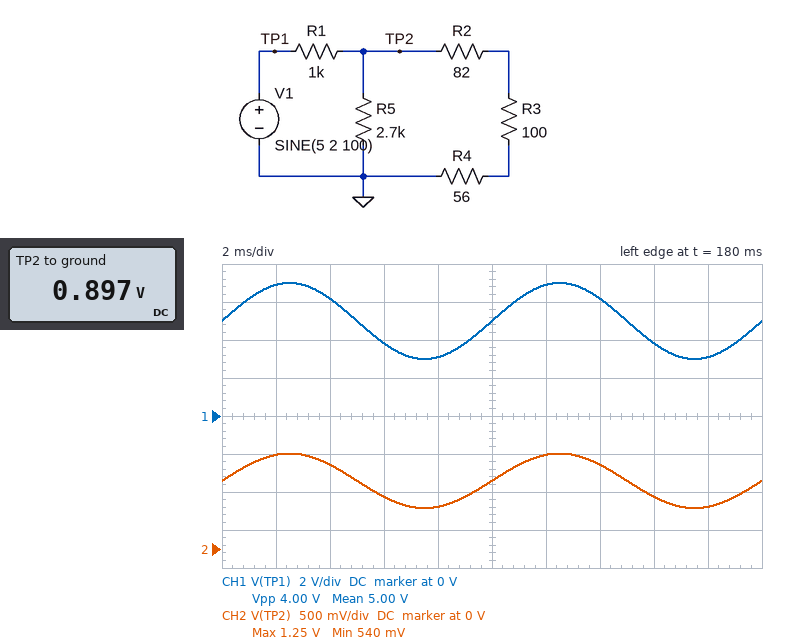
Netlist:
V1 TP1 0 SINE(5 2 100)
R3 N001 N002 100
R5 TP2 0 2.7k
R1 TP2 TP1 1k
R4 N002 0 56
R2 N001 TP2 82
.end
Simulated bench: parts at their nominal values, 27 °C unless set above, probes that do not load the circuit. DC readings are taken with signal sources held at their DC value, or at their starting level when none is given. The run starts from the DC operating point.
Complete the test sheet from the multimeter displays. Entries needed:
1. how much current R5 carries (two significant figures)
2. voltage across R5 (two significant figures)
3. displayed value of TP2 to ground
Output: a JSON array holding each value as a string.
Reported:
["330 µA", "900 mV", "0.897 V"]
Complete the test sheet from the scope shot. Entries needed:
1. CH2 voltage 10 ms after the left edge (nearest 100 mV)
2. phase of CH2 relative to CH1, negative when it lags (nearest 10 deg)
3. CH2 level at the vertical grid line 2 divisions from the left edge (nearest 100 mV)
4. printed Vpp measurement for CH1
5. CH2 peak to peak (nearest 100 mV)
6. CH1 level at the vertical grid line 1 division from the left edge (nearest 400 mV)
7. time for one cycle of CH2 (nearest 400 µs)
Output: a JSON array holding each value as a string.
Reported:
["900 mV", "0 deg", "1.1 V", "4.00 V", "700 mV", "6.8 V", "10.0 ms"]
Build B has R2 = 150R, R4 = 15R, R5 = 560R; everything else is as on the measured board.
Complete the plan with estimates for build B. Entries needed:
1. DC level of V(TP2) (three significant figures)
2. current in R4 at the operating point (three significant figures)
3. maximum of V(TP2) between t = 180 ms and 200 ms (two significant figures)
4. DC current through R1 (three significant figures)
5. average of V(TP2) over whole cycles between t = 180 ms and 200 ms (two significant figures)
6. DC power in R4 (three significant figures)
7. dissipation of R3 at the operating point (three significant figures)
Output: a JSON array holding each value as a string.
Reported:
["762 mV", "2.88 mA", "1.1 V", "4.24 mA", "760 mV", "124 µW", "827 µW"]
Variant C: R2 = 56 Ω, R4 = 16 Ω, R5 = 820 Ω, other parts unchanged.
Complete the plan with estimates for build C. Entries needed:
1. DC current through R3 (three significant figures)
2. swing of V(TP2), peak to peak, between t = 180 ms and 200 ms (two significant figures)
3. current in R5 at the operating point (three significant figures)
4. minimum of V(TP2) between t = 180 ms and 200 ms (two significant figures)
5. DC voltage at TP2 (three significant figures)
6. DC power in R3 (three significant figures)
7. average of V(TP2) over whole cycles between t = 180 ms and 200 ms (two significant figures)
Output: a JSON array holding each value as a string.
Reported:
["3.62 mA", "500 mV", "759 µA", "370 mV", "622 mV", "1.31 mW", "620 mV"]
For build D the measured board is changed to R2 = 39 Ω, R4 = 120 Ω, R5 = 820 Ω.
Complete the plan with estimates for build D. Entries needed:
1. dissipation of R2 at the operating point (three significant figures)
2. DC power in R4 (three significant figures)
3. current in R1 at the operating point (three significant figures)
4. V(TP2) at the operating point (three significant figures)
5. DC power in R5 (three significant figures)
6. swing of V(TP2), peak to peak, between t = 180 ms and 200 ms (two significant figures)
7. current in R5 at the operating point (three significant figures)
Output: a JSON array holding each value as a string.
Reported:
["393 µW", "1.21 mW", "4.18 mA", "822 mV", "825 µW", "660 mV", "1.00 mA"]
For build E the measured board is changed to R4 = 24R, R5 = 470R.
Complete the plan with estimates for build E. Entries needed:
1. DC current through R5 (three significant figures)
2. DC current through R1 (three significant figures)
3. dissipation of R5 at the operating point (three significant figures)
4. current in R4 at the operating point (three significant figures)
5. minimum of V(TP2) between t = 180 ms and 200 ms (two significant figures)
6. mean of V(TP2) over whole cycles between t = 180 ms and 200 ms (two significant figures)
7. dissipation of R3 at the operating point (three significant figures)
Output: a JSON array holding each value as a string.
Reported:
["1.33 mA", "4.37 mA", "835 µW", "3.04 mA", "380 mV", "630 mV", "925 µW"]
